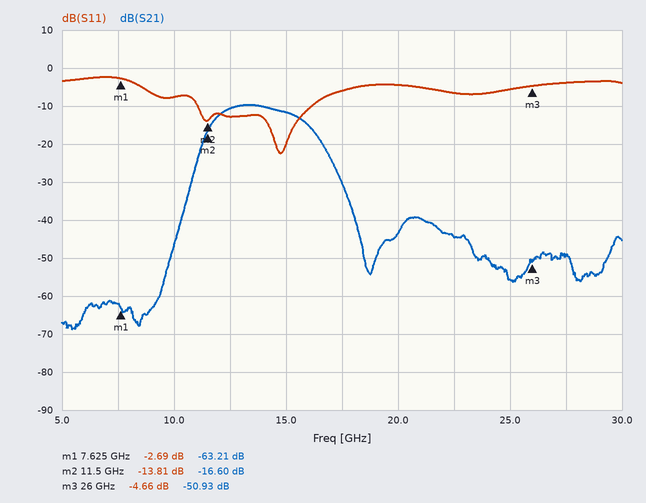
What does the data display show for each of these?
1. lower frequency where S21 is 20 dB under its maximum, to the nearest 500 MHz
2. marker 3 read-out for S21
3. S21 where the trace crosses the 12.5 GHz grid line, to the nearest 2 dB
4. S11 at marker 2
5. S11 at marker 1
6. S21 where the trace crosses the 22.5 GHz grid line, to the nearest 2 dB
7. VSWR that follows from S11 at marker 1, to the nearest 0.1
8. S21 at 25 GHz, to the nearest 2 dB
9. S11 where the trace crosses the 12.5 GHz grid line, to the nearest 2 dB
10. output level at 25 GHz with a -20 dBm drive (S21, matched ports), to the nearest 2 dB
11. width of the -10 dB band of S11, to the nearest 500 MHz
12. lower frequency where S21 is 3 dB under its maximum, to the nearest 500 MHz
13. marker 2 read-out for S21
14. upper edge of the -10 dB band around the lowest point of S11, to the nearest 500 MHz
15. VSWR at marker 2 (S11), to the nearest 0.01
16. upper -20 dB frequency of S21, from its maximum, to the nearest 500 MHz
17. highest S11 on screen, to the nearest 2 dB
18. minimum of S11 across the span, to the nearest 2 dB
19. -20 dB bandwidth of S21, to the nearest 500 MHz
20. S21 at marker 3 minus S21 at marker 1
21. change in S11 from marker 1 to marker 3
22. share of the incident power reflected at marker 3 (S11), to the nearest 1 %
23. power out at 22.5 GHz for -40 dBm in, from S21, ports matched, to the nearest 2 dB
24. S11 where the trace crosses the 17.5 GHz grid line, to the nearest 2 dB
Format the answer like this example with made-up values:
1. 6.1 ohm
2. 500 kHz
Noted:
1. 11.0 GHz
2. -50.93 dB
3. -10 dB
4. -13.81 dB
5. -2.69 dB
6. -44 dB
7. 6.5
8. -56 dB
9. -12 dB
10. -76 dBm
11. 5.0 GHz
12. 12.0 GHz
13. -16.60 dB
14. 16.0 GHz
15. 1.51
16. 17.5 GHz
17. -2 dB
18. -22 dB
19. 6.5 GHz
20. 12.28 dB
21. -1.97 dB
22. 34 %
23. -84 dBm
24. -6 dB
